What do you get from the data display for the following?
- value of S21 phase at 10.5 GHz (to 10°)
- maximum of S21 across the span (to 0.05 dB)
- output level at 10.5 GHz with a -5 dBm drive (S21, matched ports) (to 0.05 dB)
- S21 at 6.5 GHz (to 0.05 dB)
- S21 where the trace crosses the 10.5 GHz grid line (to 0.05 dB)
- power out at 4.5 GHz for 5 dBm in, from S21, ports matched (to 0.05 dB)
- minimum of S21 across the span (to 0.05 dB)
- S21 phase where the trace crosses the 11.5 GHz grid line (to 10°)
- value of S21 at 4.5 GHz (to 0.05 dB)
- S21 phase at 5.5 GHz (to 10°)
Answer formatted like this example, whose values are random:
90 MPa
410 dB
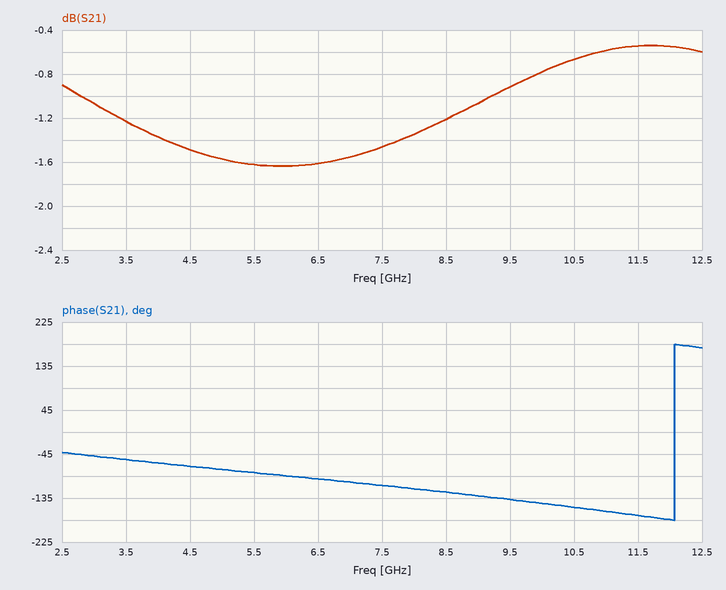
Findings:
-150°
-0.55 dB
-5.65 dBm
-1.60 dB
-0.65 dB
3.50 dBm
-1.65 dB
-170°
-1.50 dB
-80°
